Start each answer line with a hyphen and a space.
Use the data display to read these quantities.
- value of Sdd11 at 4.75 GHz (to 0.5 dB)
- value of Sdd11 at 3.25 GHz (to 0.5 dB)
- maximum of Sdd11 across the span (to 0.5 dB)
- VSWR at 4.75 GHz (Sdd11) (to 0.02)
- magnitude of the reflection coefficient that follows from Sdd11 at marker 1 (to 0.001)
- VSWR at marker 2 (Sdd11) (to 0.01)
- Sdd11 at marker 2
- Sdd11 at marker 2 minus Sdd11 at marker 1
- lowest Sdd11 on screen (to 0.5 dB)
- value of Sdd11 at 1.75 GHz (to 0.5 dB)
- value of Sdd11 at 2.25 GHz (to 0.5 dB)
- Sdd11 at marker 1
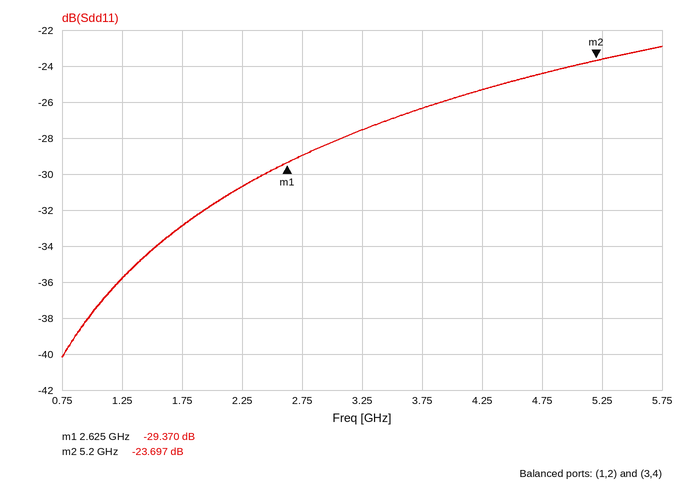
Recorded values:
- -24.5 dB
- -27.5 dB
- -23.0 dB
- 1.12
- 0.034
- 1.14
- -23.697 dB
- 5.673 dB
- -40.0 dB
- -33.0 dB
- -30.5 dB
- -29.370 dB
